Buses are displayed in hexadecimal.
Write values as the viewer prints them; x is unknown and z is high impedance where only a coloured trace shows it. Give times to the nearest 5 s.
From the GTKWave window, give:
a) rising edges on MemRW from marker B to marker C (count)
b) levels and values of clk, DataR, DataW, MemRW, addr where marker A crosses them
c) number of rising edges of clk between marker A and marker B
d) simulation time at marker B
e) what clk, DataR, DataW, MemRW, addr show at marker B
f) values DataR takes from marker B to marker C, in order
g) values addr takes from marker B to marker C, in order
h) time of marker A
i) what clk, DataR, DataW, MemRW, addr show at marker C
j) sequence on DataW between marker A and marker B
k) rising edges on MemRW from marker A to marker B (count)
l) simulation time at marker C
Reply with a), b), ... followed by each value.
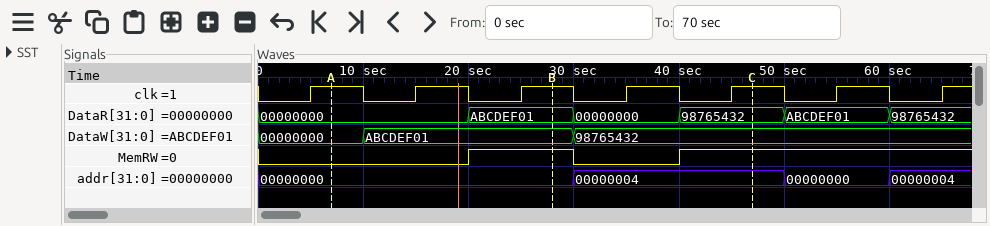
a) 1
b) clk=1, DataR=00000000, DataW=00000000, MemRW=0, addr=00000000
c) 2
d) 30 s
e) clk=1, DataR=ABCDEF01, DataW=ABCDEF01, MemRW=1, addr=00000000
f) ABCDEF01, 00000000, 98765432
g) 00000000, 00000004
h) 5 s
i) clk=1, DataR=98765432, DataW=98765432, MemRW=1, addr=00000004
j) 00000000, ABCDEF01
k) 1
l) 45 s
